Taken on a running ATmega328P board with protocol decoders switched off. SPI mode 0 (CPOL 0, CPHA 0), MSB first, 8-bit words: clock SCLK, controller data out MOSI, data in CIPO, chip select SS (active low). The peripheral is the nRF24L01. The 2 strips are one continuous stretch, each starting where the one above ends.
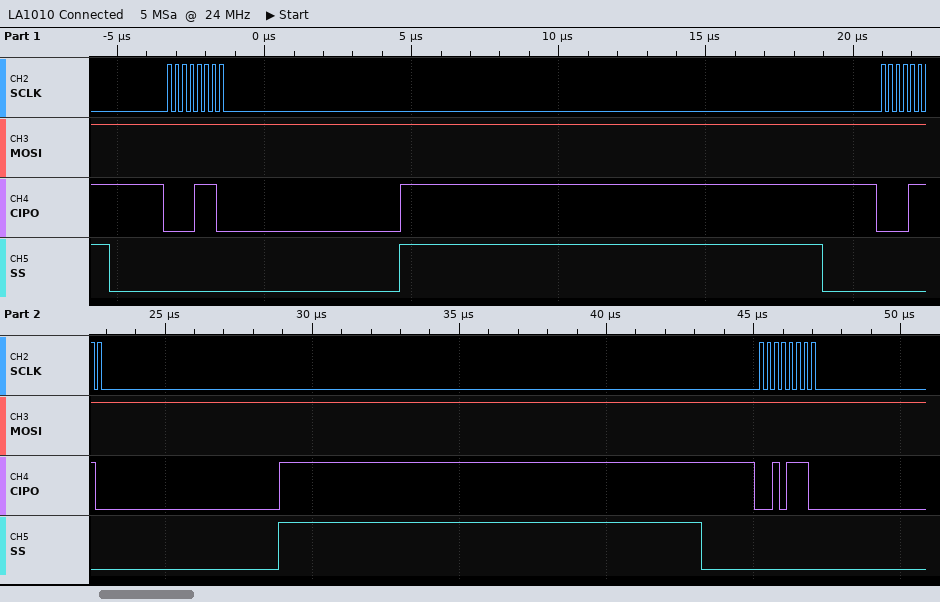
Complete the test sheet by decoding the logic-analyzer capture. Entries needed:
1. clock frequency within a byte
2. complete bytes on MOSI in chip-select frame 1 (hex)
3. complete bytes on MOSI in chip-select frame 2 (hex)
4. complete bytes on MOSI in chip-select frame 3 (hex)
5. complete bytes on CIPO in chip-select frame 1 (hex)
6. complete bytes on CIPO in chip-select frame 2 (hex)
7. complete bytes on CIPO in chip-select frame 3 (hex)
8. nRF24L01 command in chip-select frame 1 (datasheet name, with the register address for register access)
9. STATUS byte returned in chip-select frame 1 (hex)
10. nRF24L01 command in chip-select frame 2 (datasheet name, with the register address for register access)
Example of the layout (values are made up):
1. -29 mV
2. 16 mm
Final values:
1. 4 MHz
2. FF
3. FF
4. FF
5. 0E
6. 0E
7. 2E
8. NOP
9. 0x0E
10. NOP
